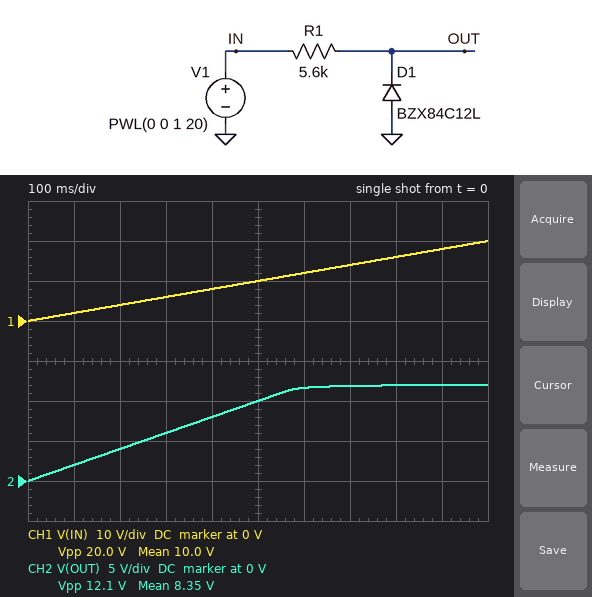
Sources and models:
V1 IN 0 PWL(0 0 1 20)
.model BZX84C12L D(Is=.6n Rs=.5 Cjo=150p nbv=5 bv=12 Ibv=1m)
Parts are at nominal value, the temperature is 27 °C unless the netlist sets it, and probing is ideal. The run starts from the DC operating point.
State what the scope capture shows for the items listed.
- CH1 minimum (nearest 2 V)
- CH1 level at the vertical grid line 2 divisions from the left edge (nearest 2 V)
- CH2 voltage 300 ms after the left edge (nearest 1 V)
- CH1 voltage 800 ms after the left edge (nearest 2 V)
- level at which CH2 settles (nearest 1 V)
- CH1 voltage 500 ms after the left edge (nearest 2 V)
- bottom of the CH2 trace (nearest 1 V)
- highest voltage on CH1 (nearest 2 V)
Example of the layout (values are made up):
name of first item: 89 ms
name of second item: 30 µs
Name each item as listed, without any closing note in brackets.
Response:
CH1 minimum: 0 V
CH1 level at the vertical grid line 2 divisions from the left edge: 4 V
CH2 voltage 300 ms after the left edge: 6 V
CH1 voltage 800 ms after the left edge: 16 V
level at which CH2 settles: 12 V
CH1 voltage 500 ms after the left edge: 10 V
bottom of the CH2 trace: 0 V
highest voltage on CH1: 20 V
